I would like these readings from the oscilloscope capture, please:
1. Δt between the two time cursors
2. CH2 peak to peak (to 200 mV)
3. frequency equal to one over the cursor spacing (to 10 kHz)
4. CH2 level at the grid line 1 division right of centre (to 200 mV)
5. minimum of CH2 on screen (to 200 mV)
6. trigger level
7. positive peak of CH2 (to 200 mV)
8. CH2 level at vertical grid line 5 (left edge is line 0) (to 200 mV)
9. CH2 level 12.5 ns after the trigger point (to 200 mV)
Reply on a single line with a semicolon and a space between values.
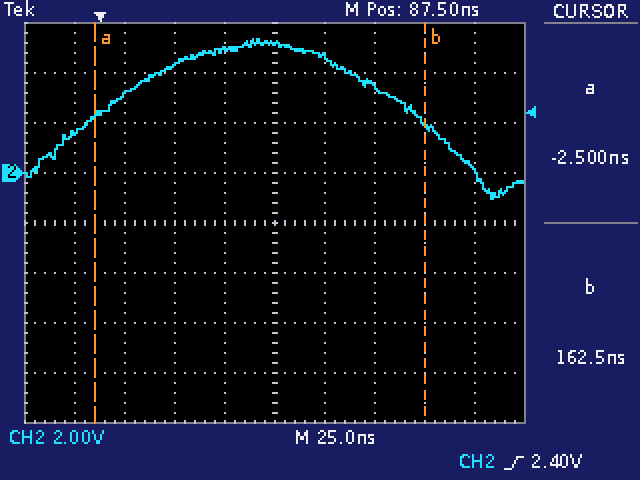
165.0 ns; 6.4 V; 6.06 MHz; 4.6 V; -1.0 V; 2.40 V; 5.4 V; 5.2 V; 3.2 V
